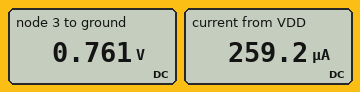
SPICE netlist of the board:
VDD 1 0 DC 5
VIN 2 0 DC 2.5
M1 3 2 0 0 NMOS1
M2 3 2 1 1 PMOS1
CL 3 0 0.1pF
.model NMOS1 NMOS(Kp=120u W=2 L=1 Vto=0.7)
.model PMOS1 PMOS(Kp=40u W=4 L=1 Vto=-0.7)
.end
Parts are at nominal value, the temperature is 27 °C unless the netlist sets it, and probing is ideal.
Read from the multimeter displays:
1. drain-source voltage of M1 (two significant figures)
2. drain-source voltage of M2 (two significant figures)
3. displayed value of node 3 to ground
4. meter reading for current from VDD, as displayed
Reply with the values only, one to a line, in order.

760 mV
-4.2 V
0.761 V
259.2 µA
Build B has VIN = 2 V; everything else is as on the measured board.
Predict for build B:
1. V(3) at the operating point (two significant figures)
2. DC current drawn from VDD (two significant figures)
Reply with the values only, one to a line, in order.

4.4 V
200 µA
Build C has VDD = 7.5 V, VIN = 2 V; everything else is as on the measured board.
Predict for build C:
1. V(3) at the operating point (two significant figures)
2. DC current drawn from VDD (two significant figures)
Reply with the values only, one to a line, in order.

7.2 V
200 µA
